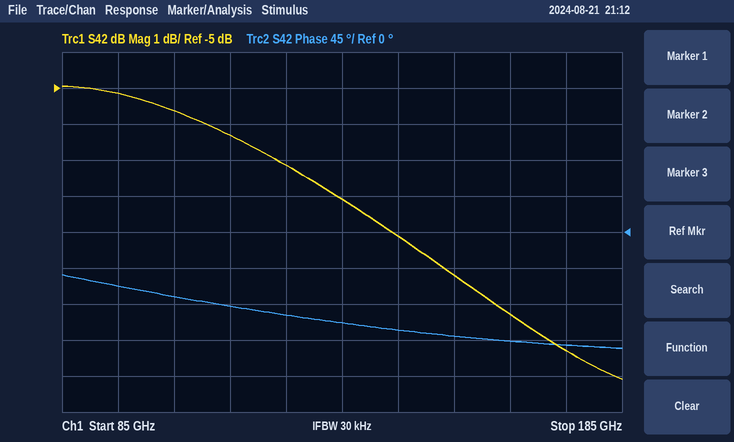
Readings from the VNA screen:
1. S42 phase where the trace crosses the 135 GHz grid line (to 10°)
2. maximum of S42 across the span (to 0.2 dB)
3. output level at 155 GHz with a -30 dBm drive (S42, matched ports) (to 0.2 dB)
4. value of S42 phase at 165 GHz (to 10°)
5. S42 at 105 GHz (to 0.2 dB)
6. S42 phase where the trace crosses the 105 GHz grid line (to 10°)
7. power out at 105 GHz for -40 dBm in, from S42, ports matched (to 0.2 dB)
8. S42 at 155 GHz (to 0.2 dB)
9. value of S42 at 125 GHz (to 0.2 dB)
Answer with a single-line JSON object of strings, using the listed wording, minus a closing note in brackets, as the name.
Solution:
{"S42 phase where the trace crosses the 135 GHz grid line": "-110°", "maximum of S42 across the span": "-5.0 dB", "output level at 155 GHz with a -30 dBm drive (S42, matched ports)": "-40.2 dBm", "value of S42 phase at 165 GHz": "-140°", "S42 at 105 GHz": "-5.6 dB", "S42 phase where the trace crosses the 105 GHz grid line": "-80°", "power out at 105 GHz for -40 dBm in, from S42, ports matched": "-45.6 dBm", "S42 at 155 GHz": "-10.2 dB", "value of S42 at 125 GHz": "-7.2 dB"}
